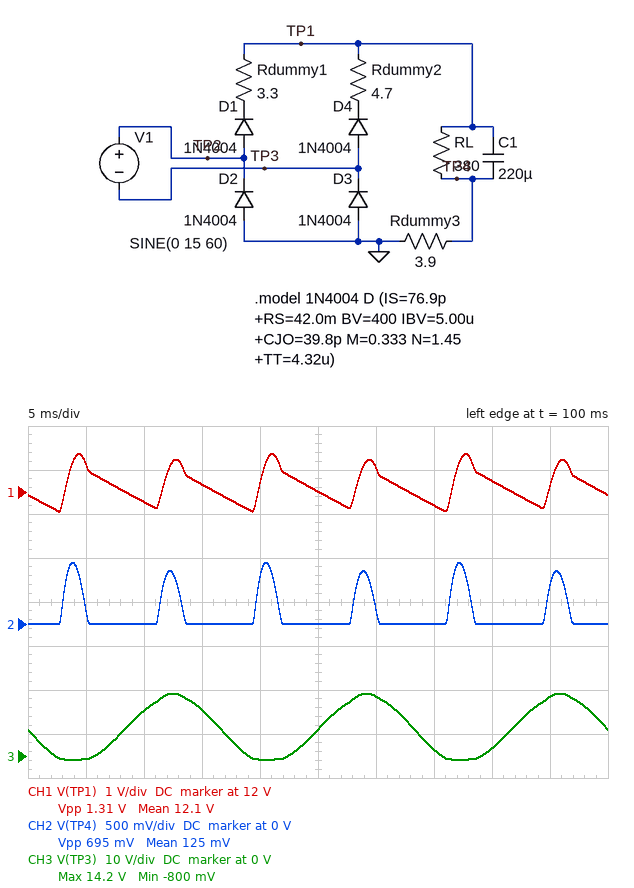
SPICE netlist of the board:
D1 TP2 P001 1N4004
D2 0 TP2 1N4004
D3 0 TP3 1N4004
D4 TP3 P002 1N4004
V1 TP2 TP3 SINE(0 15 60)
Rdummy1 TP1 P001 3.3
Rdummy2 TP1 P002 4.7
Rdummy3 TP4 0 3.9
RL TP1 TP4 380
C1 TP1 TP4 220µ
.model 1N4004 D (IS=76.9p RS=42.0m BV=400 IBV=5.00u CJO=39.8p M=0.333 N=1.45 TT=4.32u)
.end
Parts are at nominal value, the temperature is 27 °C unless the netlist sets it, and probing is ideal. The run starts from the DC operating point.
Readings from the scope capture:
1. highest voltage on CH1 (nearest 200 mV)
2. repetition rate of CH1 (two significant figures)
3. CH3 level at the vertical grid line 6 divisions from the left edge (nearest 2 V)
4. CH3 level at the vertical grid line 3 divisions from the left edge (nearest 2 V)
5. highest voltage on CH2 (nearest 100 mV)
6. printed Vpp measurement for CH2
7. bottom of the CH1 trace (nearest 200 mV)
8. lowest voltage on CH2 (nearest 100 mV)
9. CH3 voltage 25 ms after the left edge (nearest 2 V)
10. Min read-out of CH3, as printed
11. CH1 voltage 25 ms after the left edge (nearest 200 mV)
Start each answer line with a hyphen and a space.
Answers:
- 12.8 V
- 120 Hz
- 14 V
- 10 V
- 700 mV
- 695 mV
- 11.6 V
- 0 V
- 6 V
- -800 mV
- 12.0 V
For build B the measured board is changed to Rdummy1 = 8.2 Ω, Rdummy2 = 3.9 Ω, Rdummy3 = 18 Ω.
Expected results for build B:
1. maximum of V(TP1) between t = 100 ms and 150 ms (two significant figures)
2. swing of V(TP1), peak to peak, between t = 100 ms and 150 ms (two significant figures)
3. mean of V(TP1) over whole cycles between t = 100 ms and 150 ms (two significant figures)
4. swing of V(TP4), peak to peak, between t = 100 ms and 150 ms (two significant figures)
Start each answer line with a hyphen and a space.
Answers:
- 13 V
- 2.5 V
- 11 V
- 2.1 V
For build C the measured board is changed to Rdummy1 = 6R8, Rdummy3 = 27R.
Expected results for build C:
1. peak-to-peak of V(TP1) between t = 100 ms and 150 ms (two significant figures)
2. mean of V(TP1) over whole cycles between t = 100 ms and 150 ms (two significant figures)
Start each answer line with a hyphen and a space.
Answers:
- 3.0 V
- 11 V
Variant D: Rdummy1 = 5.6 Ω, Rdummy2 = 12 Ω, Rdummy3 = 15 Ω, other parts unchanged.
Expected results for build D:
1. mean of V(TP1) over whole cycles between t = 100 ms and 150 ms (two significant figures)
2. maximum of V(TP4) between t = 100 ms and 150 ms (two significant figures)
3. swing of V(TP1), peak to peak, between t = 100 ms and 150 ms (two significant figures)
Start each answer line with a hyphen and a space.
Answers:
- 11 V
- 1.9 V
- 2.3 V
